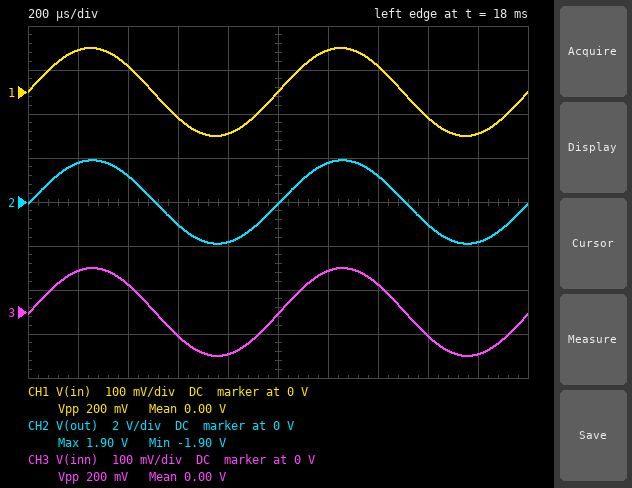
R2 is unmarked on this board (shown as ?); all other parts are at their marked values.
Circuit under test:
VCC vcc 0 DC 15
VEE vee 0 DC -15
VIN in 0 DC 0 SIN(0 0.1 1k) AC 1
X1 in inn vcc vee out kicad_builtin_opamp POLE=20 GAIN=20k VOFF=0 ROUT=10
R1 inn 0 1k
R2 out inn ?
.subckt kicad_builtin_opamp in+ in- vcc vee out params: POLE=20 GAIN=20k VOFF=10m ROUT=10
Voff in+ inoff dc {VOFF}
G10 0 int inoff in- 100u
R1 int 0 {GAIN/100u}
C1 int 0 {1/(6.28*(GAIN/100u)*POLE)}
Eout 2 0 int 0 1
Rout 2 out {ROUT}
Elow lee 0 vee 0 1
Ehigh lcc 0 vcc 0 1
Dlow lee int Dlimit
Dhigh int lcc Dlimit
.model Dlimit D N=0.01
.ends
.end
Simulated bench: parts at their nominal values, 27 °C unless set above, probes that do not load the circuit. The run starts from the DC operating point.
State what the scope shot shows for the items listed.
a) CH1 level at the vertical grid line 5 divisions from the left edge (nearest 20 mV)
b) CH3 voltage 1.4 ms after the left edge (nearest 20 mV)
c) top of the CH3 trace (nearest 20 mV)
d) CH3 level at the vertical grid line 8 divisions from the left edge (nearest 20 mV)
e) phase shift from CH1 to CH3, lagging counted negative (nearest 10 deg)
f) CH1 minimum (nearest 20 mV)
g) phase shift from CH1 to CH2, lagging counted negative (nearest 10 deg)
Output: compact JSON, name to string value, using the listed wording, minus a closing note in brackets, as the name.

{"CH1 level at the vertical grid line 5 divisions from the left edge": "0 V", "CH3 voltage 1.4 ms after the left edge": "60 mV", "top of the CH3 trace": "100 mV", "CH3 level at the vertical grid line 8 divisions from the left edge": "-60 mV", "phase shift from CH1 to CH3, lagging counted negative": "0 deg", "CH1 minimum": "-100 mV", "phase shift from CH1 to CH2, lagging counted negative": "0 deg"}
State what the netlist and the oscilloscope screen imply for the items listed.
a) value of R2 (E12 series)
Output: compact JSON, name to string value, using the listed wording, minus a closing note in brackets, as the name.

{"value of R2": "18 kΩ"}
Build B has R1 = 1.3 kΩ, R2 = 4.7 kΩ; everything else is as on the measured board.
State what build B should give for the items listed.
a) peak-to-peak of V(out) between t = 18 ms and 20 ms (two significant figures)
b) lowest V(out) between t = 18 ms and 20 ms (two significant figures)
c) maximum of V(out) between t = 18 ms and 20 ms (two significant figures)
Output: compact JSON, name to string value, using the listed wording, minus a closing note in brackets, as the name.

{"peak-to-peak of V(out) between t = 18 ms and 20 ms": "920 mV", "lowest V(out) between t = 18 ms and 20 ms": "-460 mV", "maximum of V(out) between t = 18 ms and 20 ms": "460 mV"}
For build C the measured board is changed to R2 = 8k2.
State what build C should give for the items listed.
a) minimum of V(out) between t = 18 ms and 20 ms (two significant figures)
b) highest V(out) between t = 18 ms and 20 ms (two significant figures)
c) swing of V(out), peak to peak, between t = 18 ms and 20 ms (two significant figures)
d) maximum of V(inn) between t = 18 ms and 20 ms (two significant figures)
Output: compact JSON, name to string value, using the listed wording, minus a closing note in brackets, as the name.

{"minimum of V(out) between t = 18 ms and 20 ms": "-920 mV", "highest V(out) between t = 18 ms and 20 ms": "920 mV", "swing of V(out), peak to peak, between t = 18 ms and 20 ms": "1.8 V", "maximum of V(inn) between t = 18 ms and 20 ms": "100 mV"}
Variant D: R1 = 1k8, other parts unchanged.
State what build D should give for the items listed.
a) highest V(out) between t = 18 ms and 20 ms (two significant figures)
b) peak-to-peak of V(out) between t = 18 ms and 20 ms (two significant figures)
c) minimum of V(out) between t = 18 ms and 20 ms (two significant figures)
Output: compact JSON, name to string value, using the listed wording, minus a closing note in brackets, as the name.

{"highest V(out) between t = 18 ms and 20 ms": "1.1 V", "peak-to-peak of V(out) between t = 18 ms and 20 ms": "2.2 V", "minimum of V(out) between t = 18 ms and 20 ms": "-1.1 V"}
